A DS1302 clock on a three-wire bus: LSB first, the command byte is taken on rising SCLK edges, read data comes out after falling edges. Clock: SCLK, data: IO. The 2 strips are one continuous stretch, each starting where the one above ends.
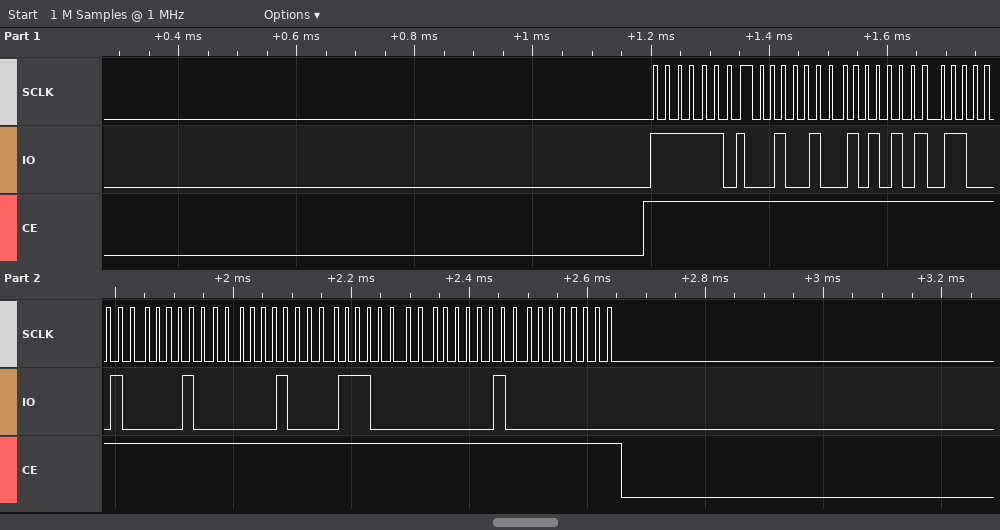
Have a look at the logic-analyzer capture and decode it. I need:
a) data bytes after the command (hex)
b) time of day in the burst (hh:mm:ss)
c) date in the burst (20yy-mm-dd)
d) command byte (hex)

24 55 23 08 08 07 20 00
23:55:24
2020-08-08
0xBF
